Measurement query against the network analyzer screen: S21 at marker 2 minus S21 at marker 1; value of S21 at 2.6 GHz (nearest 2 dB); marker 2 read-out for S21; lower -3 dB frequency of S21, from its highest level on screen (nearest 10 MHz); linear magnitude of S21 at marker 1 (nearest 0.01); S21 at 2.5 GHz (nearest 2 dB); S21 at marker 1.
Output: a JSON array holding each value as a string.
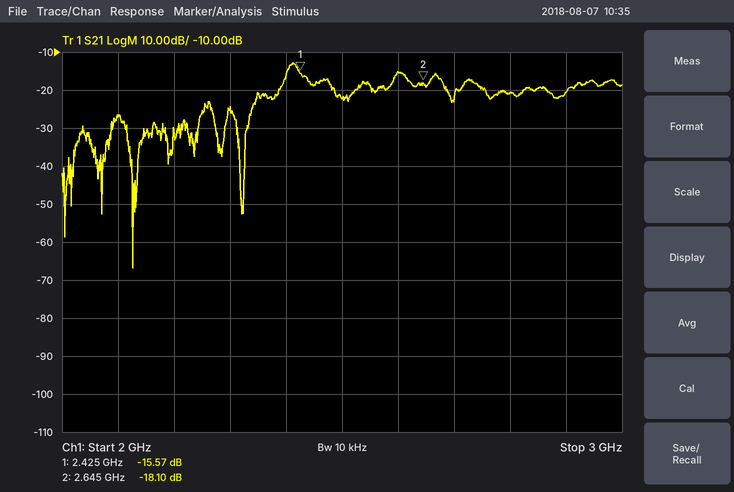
["-2.53 dB", "-16 dB", "-18.10 dB", "2.40 GHz", "0.17", "-22 dB", "-15.57 dB"]
